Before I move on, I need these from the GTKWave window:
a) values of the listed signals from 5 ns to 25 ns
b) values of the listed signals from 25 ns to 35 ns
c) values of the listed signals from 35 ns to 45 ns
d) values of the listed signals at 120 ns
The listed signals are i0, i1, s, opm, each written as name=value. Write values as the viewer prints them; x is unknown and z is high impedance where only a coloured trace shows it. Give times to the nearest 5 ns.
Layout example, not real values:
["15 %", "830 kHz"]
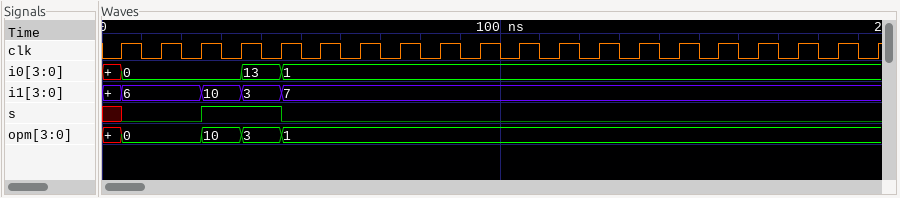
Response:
["i0=0, i1=6, s=0, opm=0", "i0=0, i1=10, s=1, opm=10", "i0=13, i1=3, s=1, opm=3", "i0=1, i1=7, s=0, opm=1"]
